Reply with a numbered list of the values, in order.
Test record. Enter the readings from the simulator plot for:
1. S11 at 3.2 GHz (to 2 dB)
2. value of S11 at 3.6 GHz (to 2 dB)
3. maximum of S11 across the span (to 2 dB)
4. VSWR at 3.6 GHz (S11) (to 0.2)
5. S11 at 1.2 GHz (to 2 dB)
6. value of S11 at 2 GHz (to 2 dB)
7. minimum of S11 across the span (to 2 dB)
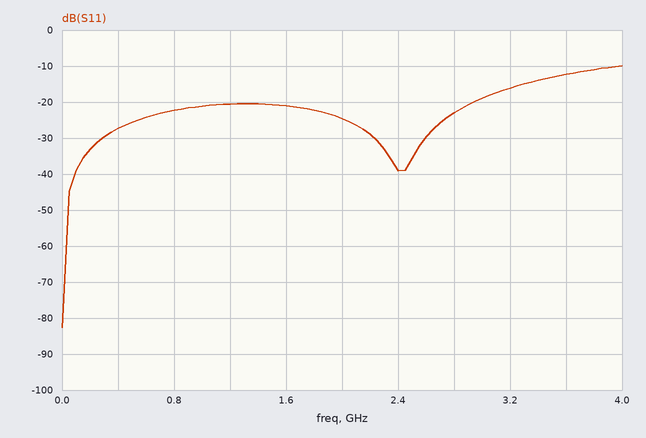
1. -16 dB
2. -12 dB
3. -10 dB
4. 1.6
5. -20 dB
6. -24 dB
7. -82 dB
